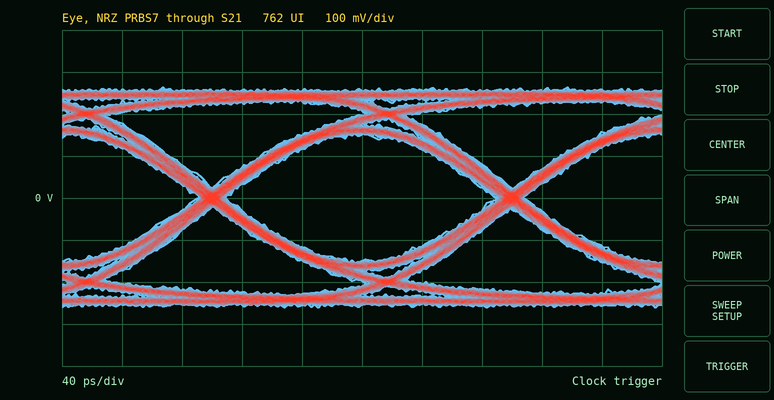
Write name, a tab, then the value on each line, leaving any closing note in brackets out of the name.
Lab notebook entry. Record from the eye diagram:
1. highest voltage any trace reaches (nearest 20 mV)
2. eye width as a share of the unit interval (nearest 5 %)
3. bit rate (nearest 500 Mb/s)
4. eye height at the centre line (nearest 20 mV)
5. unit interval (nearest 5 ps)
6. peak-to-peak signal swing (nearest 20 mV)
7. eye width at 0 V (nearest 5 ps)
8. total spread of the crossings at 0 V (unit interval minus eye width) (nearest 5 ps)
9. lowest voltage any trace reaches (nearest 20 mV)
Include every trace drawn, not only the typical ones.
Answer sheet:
highest voltage any trace reaches	260 mV
eye width as a share of the unit interval	90 %
bit rate	5.0 Gb/s
eye height at the centre line	300 mV
unit interval	200 ps
peak-to-peak signal swing	520 mV
eye width at 0 V	180 ps
total spread of the crossings at 0 V (unit interval minus eye width)	20 ps
lowest voltage any trace reaches	-260 mV
